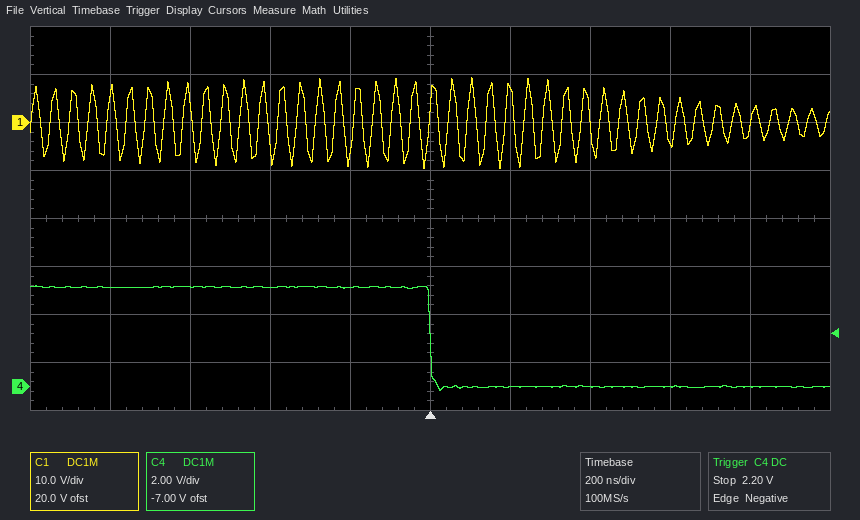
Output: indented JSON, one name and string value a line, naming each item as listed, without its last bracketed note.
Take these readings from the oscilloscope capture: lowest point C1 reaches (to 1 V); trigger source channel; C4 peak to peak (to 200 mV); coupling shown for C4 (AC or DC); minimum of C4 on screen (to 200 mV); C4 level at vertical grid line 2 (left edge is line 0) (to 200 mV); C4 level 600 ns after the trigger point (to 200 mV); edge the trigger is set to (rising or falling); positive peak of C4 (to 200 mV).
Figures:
{
  "lowest point C1 reaches": "-10 V",
  "trigger source channel": "C4",
  "C4 peak to peak": "4.4 V",
  "coupling shown for C4": "DC",
  "minimum of C4 on screen": "-200 mV",
  "C4 level at vertical grid line 2 (left edge is line 0)": "4.2 V",
  "C4 level 600 ns after the trigger point": "0.0 V",
  "edge the trigger is set to": "falling",
  "positive peak of C4": "4.2 V"
}
